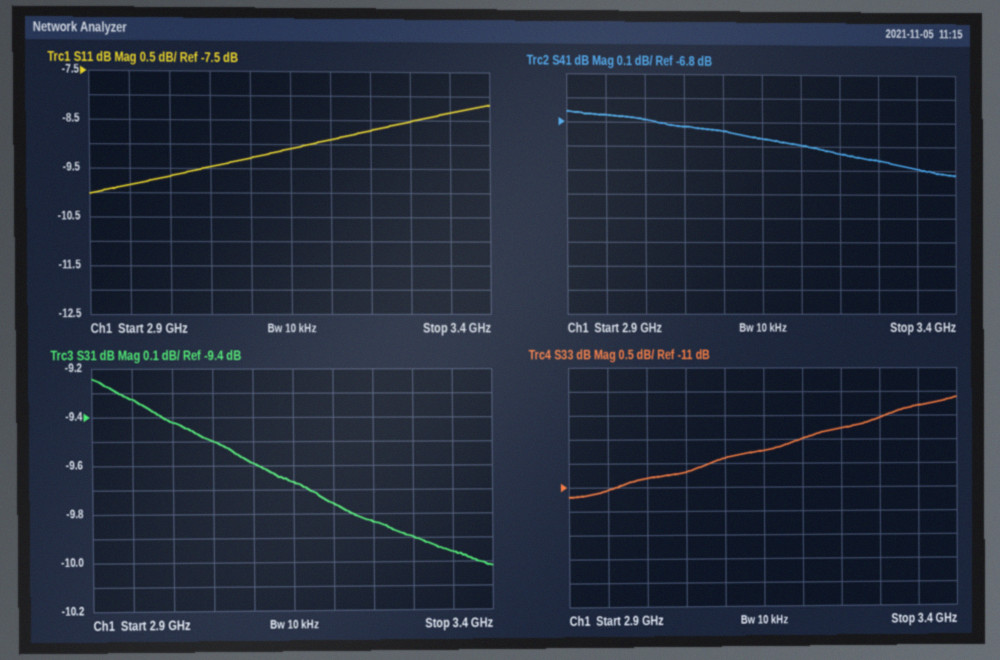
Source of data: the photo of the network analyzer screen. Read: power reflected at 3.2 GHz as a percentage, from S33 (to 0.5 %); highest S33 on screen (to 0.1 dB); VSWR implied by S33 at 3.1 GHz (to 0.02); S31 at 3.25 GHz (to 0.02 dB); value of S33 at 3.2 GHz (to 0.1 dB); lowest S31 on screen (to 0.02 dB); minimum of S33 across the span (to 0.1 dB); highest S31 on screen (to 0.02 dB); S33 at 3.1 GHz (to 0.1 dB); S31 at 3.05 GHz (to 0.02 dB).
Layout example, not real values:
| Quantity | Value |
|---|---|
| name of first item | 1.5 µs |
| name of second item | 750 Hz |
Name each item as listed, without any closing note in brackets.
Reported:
| Quantity | Value |
|---|---|
| power reflected at 3.2 GHz as a percentage, from S33 | 10.0 % |
| highest S33 on screen | -9.1 dB |
| VSWR implied by S33 at 3.1 GHz | 1.86 |
| S31 at 3.25 GHz | -9.84 dB |
| value of S33 at 3.2 GHz | -10.0 dB |
| lowest S31 on screen | -10.02 dB |
| minimum of S33 across the span | -11.2 dB |
| highest S31 on screen | -9.24 dB |
| S33 at 3.1 GHz | -10.4 dB |
| S31 at 3.05 GHz | -9.50 dB |
